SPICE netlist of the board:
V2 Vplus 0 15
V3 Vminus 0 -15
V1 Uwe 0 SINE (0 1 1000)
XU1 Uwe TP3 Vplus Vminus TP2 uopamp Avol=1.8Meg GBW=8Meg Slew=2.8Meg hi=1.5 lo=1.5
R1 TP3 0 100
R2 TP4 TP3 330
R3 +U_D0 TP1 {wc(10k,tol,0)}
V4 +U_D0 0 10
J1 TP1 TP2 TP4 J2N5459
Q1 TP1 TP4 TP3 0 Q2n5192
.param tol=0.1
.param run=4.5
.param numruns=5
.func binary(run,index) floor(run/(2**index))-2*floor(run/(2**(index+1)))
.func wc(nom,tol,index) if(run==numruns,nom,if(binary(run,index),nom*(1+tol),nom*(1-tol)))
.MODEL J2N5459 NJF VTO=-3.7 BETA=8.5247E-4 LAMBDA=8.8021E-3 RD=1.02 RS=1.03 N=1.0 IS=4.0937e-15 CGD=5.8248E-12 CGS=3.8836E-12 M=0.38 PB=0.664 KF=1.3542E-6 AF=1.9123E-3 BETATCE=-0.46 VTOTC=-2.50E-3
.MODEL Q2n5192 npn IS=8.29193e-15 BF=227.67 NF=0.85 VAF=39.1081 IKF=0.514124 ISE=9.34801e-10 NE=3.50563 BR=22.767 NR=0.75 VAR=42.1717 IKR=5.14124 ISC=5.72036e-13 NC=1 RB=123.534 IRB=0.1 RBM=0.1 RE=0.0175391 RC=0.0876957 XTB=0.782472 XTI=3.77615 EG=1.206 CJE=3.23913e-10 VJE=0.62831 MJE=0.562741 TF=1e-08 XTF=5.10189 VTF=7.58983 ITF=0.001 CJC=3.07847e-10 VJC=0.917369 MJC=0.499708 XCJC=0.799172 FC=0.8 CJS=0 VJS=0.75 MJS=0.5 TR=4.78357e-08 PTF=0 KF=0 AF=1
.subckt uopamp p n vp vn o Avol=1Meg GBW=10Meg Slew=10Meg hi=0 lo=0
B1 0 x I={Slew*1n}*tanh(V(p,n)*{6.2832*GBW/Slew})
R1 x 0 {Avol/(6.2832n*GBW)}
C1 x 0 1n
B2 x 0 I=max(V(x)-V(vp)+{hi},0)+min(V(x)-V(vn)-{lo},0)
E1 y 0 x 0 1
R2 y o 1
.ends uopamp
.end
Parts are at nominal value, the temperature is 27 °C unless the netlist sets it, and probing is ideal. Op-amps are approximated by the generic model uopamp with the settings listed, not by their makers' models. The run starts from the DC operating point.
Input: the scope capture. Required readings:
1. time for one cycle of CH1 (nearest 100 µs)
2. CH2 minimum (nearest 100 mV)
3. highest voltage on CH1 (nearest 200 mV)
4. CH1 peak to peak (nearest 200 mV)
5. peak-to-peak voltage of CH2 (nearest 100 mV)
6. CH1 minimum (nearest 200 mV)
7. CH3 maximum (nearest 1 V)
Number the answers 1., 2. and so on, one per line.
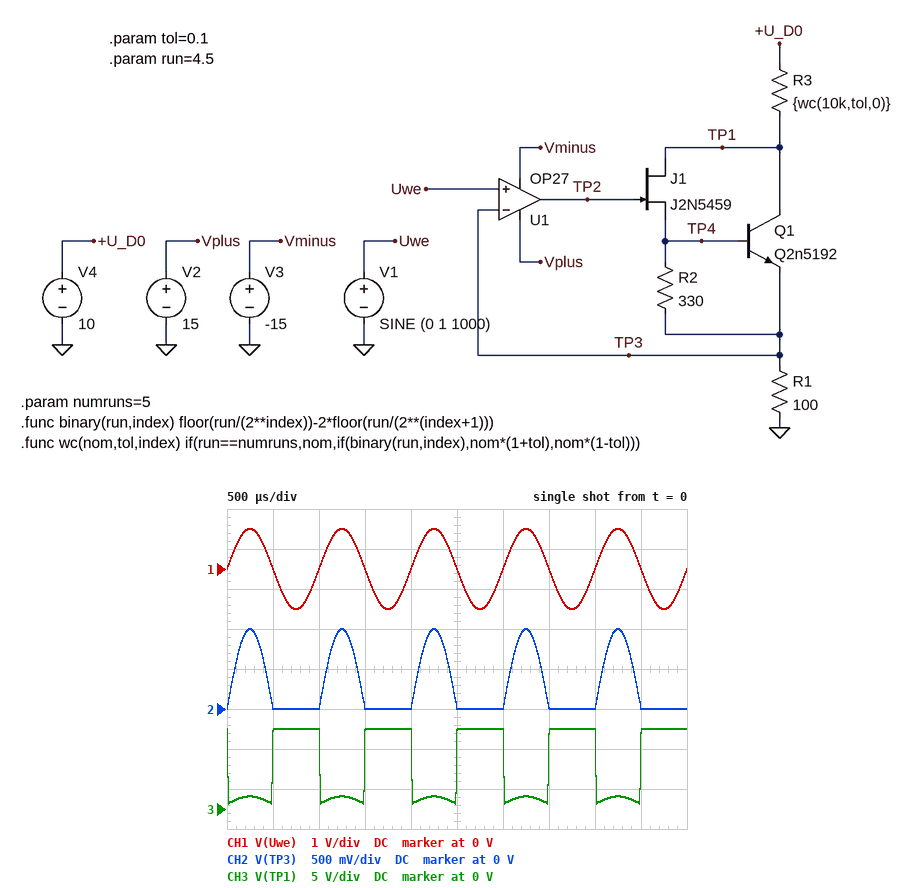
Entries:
1. 1.0 ms
2. 0 V
3. 1.0 V
4. 2.0 V
5. 1.0 V
6. -1.0 V
7. 10 V
